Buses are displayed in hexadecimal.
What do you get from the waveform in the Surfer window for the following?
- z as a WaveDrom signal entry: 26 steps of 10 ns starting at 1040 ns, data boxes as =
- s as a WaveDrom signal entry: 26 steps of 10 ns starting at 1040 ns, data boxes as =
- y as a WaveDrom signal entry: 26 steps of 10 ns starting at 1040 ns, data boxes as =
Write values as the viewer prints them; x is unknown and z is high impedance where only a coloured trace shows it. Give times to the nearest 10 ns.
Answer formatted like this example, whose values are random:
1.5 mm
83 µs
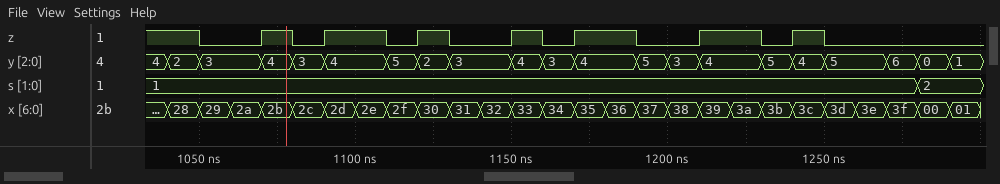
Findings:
{name: 'z', wave: '10.101.010.101.0.1.010....'}
{name: 's', wave: '=.......................=.', data: '1 2'}
{name: 'y', wave: '==.===.===.===.===.===.===', data: '2 3 4 3 4 5 2 3 4 3 4 5 3 4 5 4 5 6 0 1'}
